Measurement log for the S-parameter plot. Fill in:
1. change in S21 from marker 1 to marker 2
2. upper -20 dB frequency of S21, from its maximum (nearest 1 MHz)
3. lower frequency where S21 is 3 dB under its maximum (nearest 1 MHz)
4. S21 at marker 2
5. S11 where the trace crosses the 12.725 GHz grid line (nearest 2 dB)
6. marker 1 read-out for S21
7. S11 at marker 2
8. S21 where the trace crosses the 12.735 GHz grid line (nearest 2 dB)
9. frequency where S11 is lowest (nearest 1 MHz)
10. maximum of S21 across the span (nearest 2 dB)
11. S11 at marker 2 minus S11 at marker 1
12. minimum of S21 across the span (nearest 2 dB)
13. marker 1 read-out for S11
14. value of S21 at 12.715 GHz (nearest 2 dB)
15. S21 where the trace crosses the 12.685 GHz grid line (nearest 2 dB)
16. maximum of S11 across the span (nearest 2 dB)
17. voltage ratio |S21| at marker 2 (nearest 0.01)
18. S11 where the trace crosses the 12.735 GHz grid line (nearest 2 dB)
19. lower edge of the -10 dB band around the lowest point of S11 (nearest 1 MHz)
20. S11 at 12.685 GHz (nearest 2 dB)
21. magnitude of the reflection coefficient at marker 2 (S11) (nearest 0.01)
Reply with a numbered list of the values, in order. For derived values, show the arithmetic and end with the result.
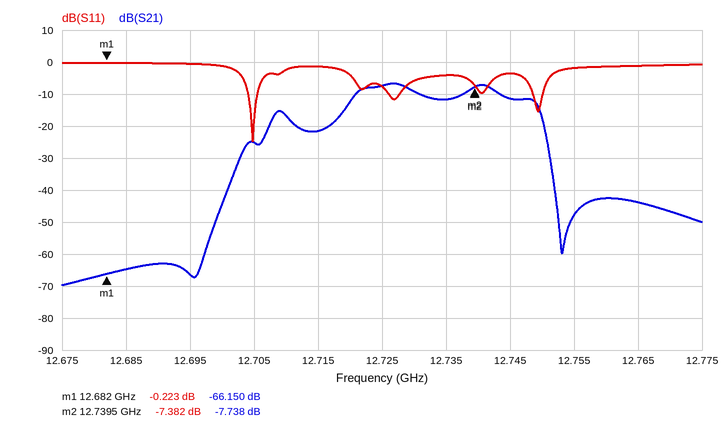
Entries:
1. -7.738 − (-66.15) = 58.412 dB
2. 12.751 GHz
3. 12.721 GHz
4. -7.738 dB
5. -8 dB
6. -66.150 dB
7. -7.382 dB
8. -12 dB
9. 12.705 GHz
10. -6 dB
11. -7.382 − (-0.223) = -7.159 dB
12. -70 dB
13. -0.223 dB
14. -22 dB
15. -64 dB
16. 0 dB
17. 10^(-7.738/20) ≈ 0.41
18. -4 dB
19. 12.704 GHz
20. 0 dB
21. 10^(-7.382/20) ≈ 0.43
